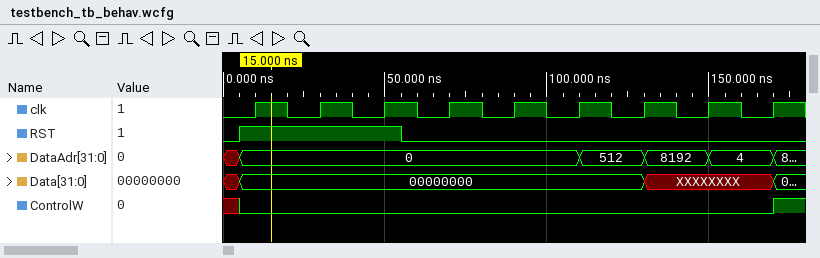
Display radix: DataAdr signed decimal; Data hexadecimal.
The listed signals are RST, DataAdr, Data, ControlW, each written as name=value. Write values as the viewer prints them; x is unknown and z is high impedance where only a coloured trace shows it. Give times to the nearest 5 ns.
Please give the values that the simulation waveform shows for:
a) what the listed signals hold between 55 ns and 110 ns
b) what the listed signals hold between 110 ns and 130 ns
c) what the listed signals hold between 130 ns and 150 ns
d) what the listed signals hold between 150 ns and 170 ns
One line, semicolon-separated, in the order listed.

RST=0, DataAdr=0, Data=00000000, ControlW=0; RST=0, DataAdr=512, Data=00000000, ControlW=0; RST=0, DataAdr=8192, Data=XXXXXXXX, ControlW=0; RST=0, DataAdr=4, Data=XXXXXXXX, ControlW=0
